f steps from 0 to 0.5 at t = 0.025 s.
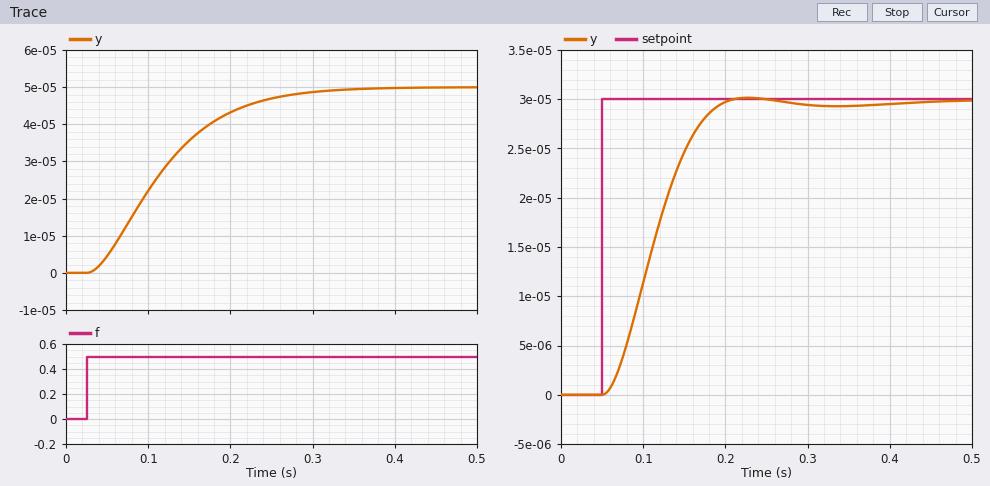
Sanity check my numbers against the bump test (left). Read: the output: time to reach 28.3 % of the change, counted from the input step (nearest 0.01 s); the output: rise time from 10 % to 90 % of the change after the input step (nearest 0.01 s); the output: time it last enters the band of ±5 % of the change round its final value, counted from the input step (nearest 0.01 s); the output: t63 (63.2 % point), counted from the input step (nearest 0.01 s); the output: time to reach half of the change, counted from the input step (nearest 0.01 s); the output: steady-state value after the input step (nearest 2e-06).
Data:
0.05 s
0.17 s
0.24 s
0.11 s
0.08 s
0.000050
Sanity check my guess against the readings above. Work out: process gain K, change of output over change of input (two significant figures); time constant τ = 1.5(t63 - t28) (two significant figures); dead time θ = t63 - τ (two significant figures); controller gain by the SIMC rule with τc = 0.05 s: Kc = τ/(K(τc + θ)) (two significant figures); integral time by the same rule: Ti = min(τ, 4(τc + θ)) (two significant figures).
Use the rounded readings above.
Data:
0.00010
0.090 s
0.020 s
13000
0.090 s
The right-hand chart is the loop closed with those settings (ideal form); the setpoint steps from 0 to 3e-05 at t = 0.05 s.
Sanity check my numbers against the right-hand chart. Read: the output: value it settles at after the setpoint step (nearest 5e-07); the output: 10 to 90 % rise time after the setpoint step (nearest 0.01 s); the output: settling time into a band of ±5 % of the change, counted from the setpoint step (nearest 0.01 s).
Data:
0.0000300
0.09 s
0.13 s
